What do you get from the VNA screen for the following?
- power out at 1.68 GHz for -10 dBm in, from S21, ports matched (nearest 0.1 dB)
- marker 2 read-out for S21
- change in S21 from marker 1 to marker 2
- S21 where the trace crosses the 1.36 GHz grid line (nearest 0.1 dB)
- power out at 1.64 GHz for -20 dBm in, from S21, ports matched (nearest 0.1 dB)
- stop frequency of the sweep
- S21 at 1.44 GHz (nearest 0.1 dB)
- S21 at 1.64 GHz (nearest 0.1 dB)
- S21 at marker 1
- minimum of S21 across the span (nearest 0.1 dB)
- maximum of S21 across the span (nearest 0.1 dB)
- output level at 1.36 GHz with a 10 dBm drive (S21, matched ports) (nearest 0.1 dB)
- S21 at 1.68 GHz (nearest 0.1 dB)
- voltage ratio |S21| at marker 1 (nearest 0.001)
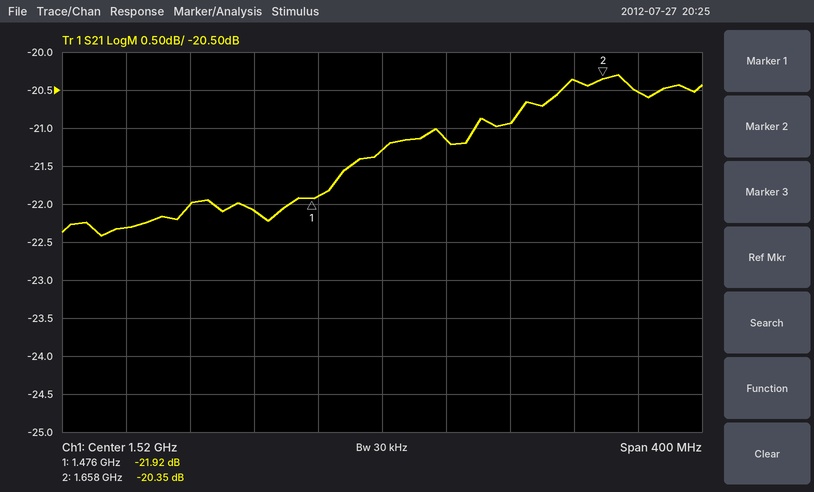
-30.5 dBm
-20.35 dB
1.57 dB
-22.3 dB
-40.4 dBm
1.72 GHz
-22.1 dB
-20.4 dB
-21.92 dB
-22.4 dB
-20.3 dB
-12.3 dBm
-20.5 dB
0.080
